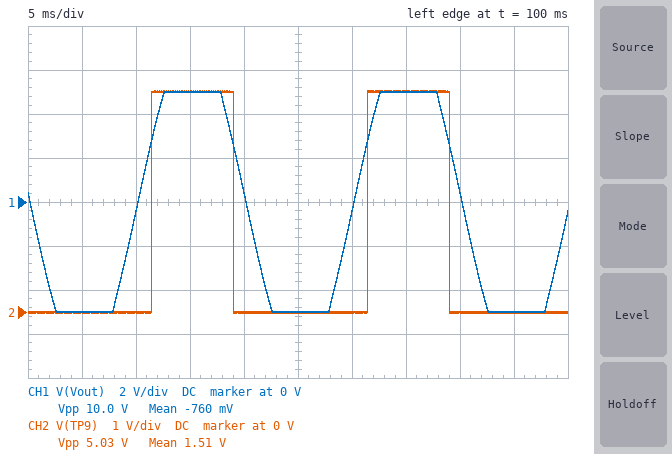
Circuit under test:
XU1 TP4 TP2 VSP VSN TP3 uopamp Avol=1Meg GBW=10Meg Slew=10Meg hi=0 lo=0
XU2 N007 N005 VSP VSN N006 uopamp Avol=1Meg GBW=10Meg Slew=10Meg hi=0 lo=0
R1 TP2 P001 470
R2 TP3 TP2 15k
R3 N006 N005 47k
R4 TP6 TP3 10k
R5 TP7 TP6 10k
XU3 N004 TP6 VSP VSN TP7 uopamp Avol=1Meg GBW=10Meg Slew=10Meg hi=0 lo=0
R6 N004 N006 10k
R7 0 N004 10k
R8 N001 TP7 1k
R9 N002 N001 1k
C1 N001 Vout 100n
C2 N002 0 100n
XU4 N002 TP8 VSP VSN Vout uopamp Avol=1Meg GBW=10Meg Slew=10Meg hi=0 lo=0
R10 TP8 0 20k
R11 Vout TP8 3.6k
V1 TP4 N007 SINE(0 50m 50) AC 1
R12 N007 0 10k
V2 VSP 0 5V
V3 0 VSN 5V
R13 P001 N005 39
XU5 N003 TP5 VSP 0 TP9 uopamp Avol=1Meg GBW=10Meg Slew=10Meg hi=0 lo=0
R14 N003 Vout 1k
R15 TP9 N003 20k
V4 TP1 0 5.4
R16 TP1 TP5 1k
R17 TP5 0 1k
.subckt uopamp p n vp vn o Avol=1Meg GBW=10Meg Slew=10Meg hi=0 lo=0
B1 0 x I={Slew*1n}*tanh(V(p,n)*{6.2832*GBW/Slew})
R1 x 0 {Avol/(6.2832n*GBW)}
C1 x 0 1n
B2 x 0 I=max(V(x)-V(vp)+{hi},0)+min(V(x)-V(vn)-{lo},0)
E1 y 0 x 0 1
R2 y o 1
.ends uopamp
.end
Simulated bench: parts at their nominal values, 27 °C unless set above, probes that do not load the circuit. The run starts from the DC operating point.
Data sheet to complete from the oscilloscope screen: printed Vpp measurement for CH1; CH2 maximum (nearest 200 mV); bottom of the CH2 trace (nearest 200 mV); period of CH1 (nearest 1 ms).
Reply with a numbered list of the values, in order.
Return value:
1. 10.0 V
2. 5.0 V
3. 0 V
4. 20 ms
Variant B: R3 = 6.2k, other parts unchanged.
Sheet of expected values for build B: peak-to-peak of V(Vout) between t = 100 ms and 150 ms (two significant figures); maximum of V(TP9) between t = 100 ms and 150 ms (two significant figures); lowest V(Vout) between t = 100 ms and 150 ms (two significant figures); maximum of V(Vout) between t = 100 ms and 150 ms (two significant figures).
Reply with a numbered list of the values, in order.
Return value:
1. 5.0 V
2. -9.5 mV
3. -2.5 V
4. 2.5 V
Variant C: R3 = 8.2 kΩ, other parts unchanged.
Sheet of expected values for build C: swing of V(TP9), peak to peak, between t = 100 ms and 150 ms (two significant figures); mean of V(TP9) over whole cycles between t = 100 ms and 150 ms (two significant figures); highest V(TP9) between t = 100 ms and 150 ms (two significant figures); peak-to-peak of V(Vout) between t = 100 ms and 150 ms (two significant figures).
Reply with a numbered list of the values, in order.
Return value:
1. 5.4 mV
2. -9.6 mV
3. -4.7 mV
4. 5.5 V
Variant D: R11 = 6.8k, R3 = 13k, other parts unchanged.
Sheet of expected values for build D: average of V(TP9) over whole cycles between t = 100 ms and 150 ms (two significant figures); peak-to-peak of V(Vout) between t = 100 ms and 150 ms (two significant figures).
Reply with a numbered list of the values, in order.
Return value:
1. 1.2 V
2. 7.5 V
